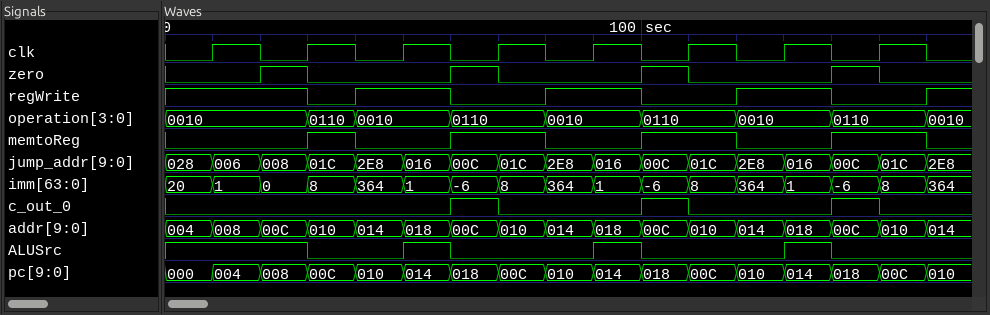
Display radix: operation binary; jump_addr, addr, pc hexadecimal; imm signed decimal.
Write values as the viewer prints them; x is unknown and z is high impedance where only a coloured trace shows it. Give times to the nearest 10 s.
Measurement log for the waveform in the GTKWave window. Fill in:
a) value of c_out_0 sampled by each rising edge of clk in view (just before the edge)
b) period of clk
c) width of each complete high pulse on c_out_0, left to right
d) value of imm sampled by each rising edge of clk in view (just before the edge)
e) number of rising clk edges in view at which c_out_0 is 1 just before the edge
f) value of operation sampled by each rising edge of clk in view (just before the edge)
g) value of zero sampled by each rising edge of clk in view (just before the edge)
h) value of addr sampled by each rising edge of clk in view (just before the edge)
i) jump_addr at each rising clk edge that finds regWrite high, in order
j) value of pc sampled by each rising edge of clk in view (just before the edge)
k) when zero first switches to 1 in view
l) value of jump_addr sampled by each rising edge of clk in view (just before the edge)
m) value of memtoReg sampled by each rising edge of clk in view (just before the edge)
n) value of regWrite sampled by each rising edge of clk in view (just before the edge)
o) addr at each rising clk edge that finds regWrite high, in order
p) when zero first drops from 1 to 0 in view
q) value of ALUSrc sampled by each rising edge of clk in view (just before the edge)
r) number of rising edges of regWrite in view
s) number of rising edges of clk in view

0 0 0 1 0 1 0 1
20 s
10 s, 10 s, 10 s
20, 0, 364, -6, 364, -6, 364, -6
3
0010, 0010, 0010, 0110, 0010, 0110, 0010, 0110
0 1 0 1 0 1 0 1
004, 00C, 014, 00C, 014, 00C, 014, 00C
028, 008, 2E8, 2E8, 2E8
000, 008, 010, 018, 010, 018, 010, 018
20 s
028, 008, 2E8, 00C, 2E8, 00C, 2E8, 00C
0 0 0 1 0 1 0 1
1 1 1 0 1 0 1 0
004, 00C, 014, 014, 014
30 s
1 1 0 0 0 0 0 0
4
8
